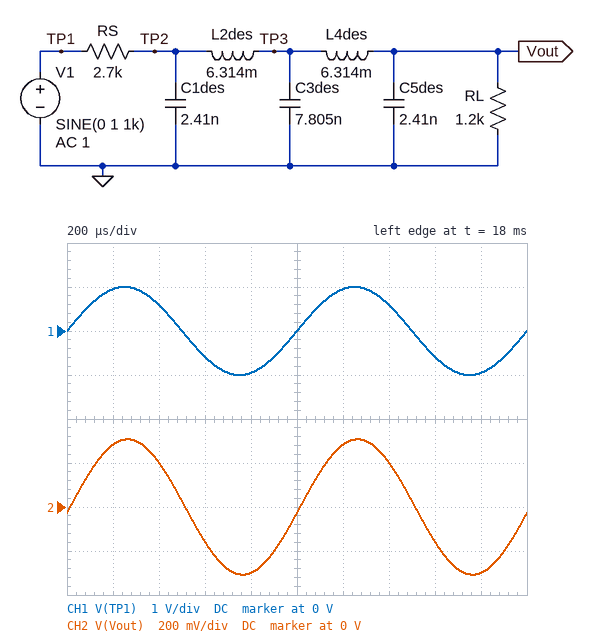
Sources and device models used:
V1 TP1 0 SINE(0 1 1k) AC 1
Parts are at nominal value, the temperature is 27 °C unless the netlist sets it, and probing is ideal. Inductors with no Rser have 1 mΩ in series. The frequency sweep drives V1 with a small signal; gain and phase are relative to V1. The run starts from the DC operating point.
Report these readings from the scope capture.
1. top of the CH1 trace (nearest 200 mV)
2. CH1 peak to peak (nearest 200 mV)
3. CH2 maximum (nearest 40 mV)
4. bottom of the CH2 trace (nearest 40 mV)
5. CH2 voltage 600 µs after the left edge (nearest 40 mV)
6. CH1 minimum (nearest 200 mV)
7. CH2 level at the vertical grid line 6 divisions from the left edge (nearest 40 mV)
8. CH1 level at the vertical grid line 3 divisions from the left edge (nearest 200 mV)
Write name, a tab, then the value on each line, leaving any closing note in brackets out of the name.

top of the CH1 trace	1.0 V
CH1 peak to peak	2.0 V
CH2 maximum	320 mV
bottom of the CH2 trace	-320 mV
CH2 voltage 600 µs after the left edge	-160 mV
CH1 minimum	-1.0 V
CH2 level at the vertical grid line 6 divisions from the left edge	280 mV
CH1 level at the vertical grid line 3 divisions from the left edge	-600 mV
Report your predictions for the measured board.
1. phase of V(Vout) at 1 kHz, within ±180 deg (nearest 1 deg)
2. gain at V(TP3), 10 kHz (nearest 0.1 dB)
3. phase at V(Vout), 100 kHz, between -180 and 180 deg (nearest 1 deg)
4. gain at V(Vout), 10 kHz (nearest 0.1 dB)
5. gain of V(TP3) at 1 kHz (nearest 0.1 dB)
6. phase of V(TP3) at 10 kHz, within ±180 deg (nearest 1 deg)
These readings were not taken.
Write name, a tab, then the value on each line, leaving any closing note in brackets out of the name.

phase of V(Vout) at 1 kHz, within ±180 deg	-5 deg
gain at V(TP3), 10 kHz	-10.7 dB
phase at V(Vout), 100 kHz, between -180 and 180 deg	-40 deg
gain at V(Vout), 10 kHz	-10.6 dB
gain of V(TP3) at 1 kHz	-10.2 dB
phase of V(TP3) at 10 kHz, within ±180 deg	-29 deg
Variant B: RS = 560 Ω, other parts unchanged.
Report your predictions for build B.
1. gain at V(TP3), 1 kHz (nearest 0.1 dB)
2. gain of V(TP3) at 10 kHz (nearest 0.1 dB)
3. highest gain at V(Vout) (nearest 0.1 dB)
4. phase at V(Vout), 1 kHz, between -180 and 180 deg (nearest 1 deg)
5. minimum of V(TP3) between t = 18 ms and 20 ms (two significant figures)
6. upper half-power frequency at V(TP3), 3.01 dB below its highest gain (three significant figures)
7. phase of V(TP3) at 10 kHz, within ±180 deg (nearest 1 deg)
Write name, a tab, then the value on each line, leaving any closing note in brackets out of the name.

gain at V(TP3), 1 kHz	-3.3 dB
gain of V(TP3) at 10 kHz	-3.1 dB
highest gain at V(Vout)	-2.8 dB
phase at V(Vout), 1 kHz, between -180 and 180 deg	-4 deg
minimum of V(TP3) between t = 18 ms and 20 ms	-680 mV
upper half-power frequency at V(TP3), 3.01 dB below its highest gain	43.4 kHz
phase of V(TP3) at 10 kHz, within ±180 deg	-25 deg
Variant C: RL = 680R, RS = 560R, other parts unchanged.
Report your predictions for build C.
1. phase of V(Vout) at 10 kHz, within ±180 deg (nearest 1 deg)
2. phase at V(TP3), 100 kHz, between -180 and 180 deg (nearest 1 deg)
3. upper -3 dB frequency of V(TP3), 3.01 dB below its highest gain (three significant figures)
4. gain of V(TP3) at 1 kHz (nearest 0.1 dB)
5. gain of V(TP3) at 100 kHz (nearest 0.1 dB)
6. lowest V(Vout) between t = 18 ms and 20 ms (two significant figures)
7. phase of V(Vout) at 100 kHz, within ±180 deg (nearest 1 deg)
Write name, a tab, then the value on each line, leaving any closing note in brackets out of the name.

phase of V(Vout) at 10 kHz, within ±180 deg	-49 deg
phase at V(TP3), 100 kHz, between -180 and 180 deg	145 deg
upper -3 dB frequency of V(TP3), 3.01 dB below its highest gain	40.0 kHz
gain of V(TP3) at 1 kHz	-5.2 dB
gain of V(TP3) at 100 kHz	-26.5 dB
lowest V(Vout) between t = 18 ms and 20 ms	-550 mV
phase of V(Vout) at 100 kHz, within ±180 deg	15 deg
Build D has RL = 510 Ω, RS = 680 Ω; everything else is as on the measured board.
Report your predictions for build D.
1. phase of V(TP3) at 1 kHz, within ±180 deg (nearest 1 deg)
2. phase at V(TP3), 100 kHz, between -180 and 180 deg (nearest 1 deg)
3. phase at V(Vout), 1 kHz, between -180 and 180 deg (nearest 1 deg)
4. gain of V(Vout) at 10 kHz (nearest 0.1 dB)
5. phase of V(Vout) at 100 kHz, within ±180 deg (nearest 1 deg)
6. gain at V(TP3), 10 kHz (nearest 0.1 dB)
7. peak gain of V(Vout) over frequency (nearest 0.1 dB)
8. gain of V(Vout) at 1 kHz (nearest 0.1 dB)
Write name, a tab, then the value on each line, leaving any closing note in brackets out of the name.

phase of V(TP3) at 1 kHz, within ±180 deg	-1 deg
phase at V(TP3), 100 kHz, between -180 and 180 deg	140 deg
phase at V(Vout), 1 kHz, between -180 and 180 deg	-5 deg
gain of V(Vout) at 10 kHz	-7.9 dB
phase of V(Vout) at 100 kHz, within ±180 deg	17 deg
gain at V(TP3), 10 kHz	-6.2 dB
peak gain of V(Vout) over frequency	-7.3 dB
gain of V(Vout) at 1 kHz	-7.4 dB
